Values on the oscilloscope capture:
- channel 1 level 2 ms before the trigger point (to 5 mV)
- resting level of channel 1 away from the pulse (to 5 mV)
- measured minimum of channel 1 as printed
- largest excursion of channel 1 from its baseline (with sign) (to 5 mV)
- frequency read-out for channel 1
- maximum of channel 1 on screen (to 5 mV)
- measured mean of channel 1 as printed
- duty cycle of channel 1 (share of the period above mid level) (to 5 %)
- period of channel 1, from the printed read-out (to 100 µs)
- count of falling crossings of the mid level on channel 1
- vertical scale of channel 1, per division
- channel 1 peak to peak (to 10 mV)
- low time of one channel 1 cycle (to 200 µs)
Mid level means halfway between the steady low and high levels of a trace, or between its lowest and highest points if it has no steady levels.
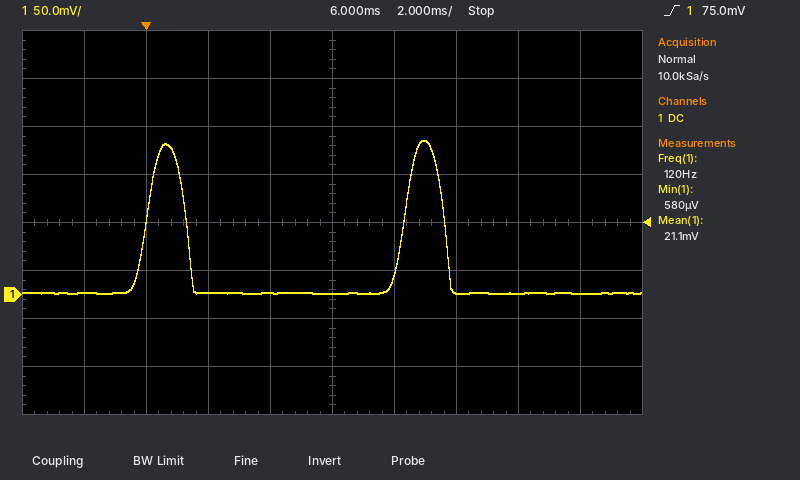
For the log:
0 mV
0 mV
580 µV
+160 mV
120 Hz
160 mV
21.1 mV
15 %
8.3 ms
2
50 mV
160 mV
7.0 ms
